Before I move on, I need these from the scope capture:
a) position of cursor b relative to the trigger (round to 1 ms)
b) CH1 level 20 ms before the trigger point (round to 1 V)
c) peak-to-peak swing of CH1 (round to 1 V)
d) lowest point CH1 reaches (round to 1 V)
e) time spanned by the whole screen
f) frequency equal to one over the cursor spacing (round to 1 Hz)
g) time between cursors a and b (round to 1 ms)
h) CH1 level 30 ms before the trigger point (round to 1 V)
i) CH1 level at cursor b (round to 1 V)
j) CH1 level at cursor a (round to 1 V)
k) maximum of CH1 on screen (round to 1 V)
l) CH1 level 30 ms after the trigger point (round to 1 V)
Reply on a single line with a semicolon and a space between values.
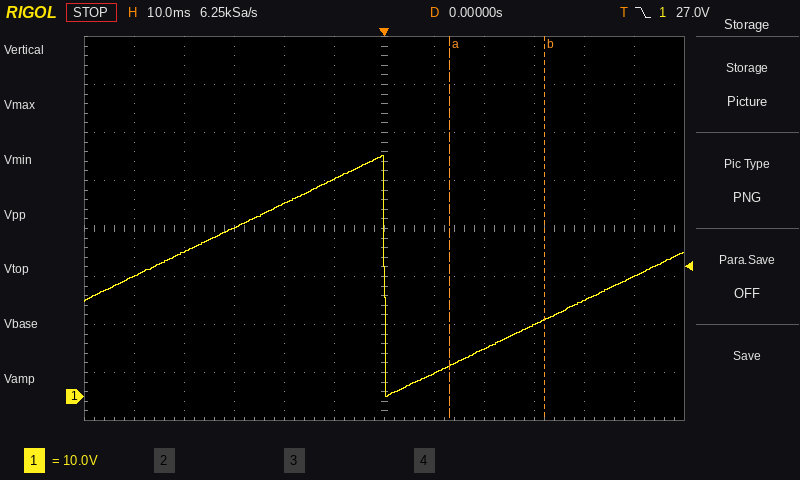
+32 ms; 40 V; 50 V; 0 V; 120 ms; 53 Hz; 19 ms; 35 V; 16 V; 6 V; 50 V; 15 V
